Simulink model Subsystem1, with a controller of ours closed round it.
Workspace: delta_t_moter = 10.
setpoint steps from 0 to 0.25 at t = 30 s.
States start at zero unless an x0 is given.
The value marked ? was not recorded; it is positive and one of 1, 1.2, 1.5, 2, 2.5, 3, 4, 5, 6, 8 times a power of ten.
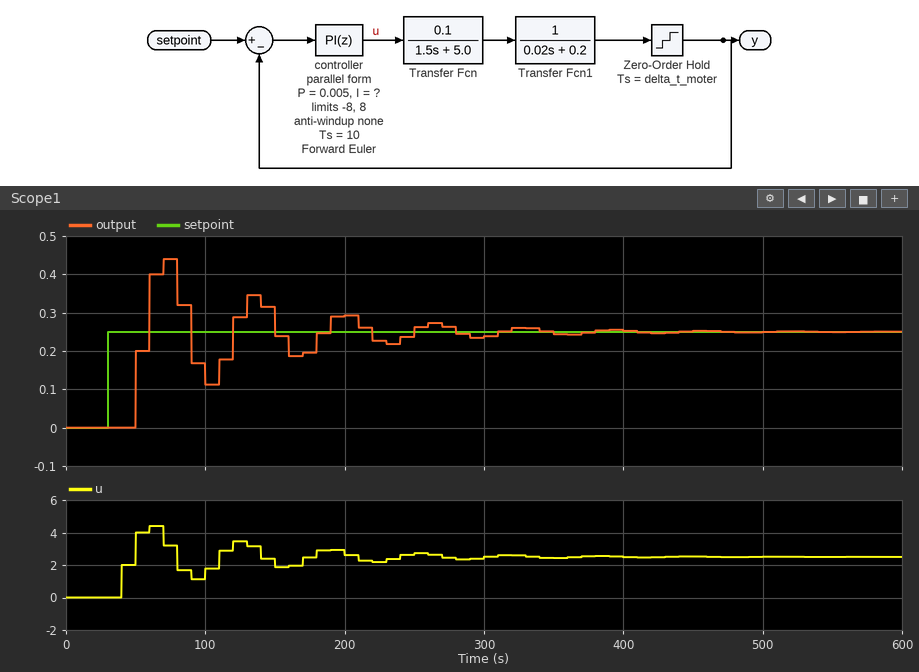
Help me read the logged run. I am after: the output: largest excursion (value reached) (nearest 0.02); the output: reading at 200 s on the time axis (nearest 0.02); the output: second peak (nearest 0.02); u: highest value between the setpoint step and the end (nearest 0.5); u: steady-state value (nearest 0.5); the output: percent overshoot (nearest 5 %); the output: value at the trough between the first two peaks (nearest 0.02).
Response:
0.44
0.30
0.34
4.5
2.5
75 %
0.12
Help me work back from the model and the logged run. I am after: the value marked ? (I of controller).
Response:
0.8
